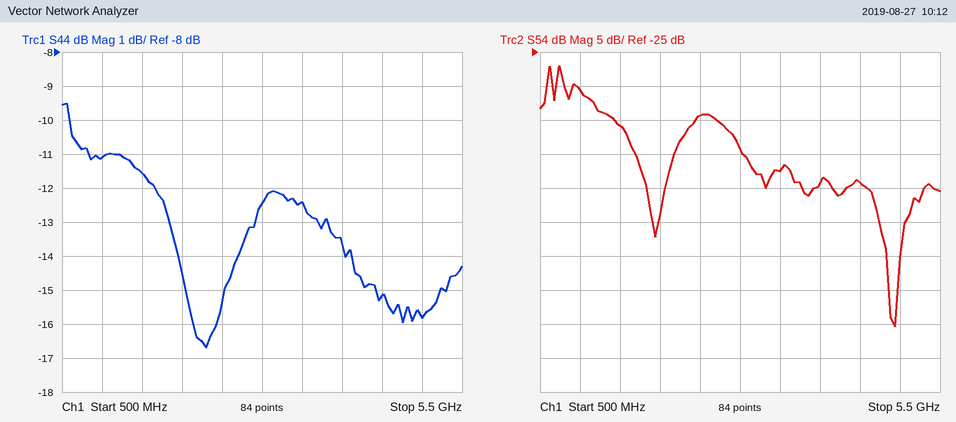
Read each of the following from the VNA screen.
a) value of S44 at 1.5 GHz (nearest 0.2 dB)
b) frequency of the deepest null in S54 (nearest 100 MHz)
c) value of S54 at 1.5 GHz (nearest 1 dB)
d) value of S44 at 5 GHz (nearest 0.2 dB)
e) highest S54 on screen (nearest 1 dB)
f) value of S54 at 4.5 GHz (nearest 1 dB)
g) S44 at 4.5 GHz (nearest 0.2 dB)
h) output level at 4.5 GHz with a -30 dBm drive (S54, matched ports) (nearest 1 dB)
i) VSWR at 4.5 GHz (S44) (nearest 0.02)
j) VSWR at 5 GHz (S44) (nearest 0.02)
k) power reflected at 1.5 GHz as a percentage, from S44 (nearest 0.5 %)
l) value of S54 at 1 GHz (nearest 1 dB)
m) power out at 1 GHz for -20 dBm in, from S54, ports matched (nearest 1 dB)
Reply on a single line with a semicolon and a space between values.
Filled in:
-11.6 dB; 4.9 GHz; -36 dB; -15.8 dB; -27 dB; -44 dB; -15.2 dB; -74 dBm; 1.42; 1.38; 7.0 %; -31 dB; -51 dBm
